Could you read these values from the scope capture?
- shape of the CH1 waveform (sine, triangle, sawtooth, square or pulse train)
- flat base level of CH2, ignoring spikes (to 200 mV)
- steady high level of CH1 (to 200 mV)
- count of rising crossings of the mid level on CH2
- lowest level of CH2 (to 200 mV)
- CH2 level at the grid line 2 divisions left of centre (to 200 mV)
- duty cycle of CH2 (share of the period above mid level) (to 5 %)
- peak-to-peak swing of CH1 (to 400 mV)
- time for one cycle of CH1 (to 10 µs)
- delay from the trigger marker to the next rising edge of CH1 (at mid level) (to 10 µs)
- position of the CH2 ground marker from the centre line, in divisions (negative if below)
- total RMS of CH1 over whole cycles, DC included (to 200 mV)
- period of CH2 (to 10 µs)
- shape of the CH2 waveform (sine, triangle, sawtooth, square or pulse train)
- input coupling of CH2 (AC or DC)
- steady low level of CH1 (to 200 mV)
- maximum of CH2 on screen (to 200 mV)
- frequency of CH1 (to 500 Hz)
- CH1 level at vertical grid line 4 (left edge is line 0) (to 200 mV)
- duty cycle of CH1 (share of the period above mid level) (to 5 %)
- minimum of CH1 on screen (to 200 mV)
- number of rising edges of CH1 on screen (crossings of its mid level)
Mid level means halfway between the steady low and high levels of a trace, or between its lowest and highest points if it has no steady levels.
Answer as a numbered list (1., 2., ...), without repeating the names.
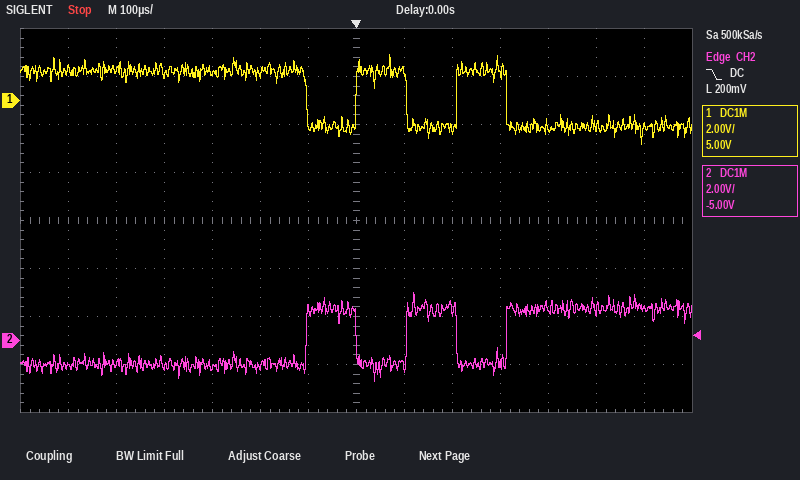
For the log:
1. square
2. -1.0 V
3. 1.2 V
4. 3
5. -1.8 V
6. -1.0 V
7. 50 %
8. 3.6 V
9. 210 µs
10. 210 µs
11. -2.5 div
12. 1.2 V
13. 210 µs
14. square
15. DC
16. -1.2 V
17. 2.0 V
18. 5.0 kHz
19. 1.2 V
20. 50 %
21. -1.8 V
22. 2
